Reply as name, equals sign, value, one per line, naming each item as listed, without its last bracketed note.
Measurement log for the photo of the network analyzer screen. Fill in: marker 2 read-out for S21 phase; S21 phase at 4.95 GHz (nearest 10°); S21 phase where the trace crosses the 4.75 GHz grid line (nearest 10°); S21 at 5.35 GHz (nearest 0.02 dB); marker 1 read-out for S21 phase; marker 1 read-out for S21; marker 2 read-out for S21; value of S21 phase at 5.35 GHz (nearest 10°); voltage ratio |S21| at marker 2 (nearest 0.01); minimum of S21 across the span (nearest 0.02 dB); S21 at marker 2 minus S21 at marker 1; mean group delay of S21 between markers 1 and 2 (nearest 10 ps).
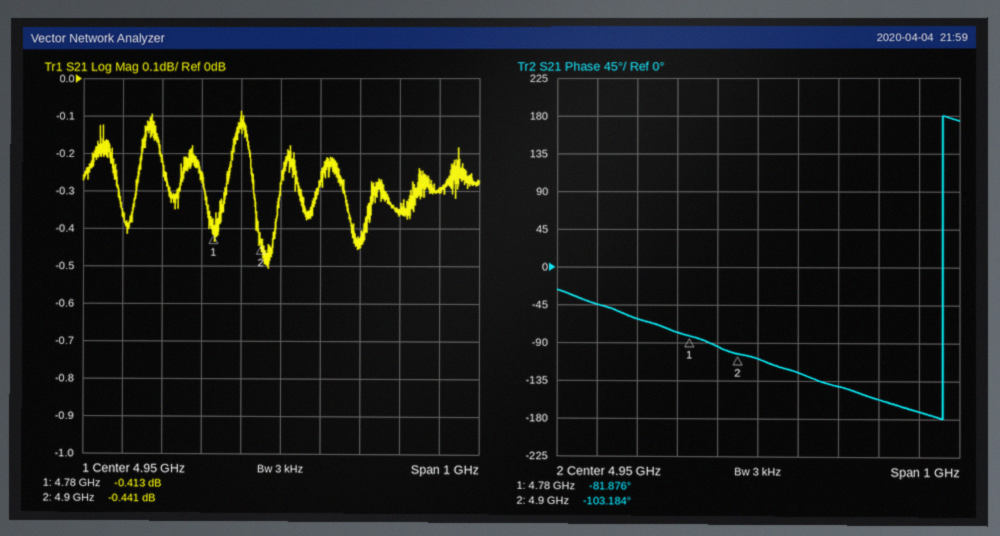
marker 2 read-out for S21 phase = -103.184°
S21 phase at 4.95 GHz = -110°
S21 phase where the trace crosses the 4.75 GHz grid line = -80°
S21 at 5.35 GHz = -0.30 dB
marker 1 read-out for S21 phase = -81.876°
marker 1 read-out for S21 = -0.413 dB
marker 2 read-out for S21 = -0.441 dB
value of S21 phase at 5.35 GHz = -170°
voltage ratio |S21| at marker 2 = 0.95
minimum of S21 across the span = -0.50 dB
S21 at marker 2 minus S21 at marker 1 = -0.028 dB
mean group delay of S21 between markers 1 and 2 = 490 ps
